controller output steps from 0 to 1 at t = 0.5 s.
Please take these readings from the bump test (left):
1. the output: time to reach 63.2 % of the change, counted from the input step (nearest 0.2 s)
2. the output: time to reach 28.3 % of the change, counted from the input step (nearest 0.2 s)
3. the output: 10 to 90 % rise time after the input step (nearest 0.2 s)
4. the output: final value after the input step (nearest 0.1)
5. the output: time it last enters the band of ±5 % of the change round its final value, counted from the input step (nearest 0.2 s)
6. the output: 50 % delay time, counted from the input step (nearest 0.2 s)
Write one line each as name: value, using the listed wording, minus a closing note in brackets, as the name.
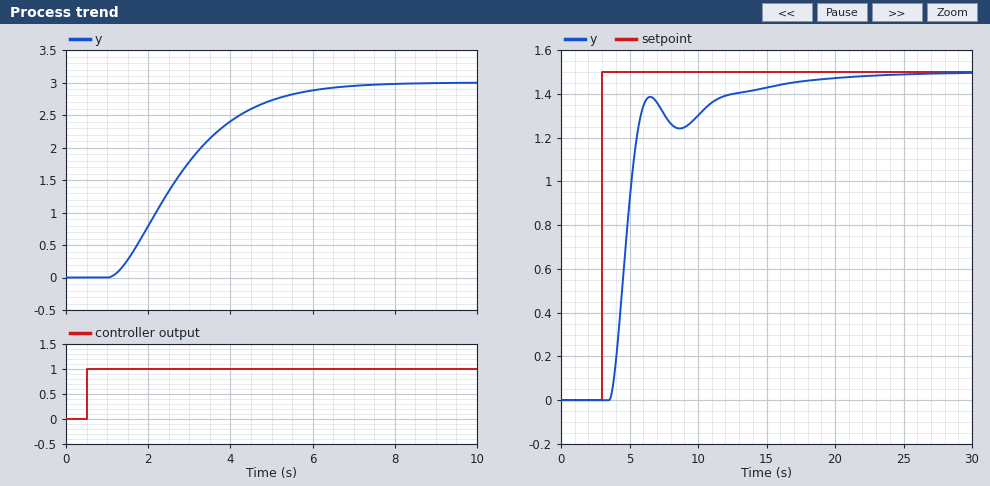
the output: time to reach 63.2 % of the change, counted from the input step: 2.6 s
the output: time to reach 28.3 % of the change, counted from the input step: 1.6 s
the output: 10 to 90 % rise time after the input step: 3.4 s
the output: final value after the input step: 3.0
the output: time it last enters the band of ±5 % of the change round its final value, counted from the input step: 5.2 s
the output: 50 % delay time, counted from the input step: 2.2 s
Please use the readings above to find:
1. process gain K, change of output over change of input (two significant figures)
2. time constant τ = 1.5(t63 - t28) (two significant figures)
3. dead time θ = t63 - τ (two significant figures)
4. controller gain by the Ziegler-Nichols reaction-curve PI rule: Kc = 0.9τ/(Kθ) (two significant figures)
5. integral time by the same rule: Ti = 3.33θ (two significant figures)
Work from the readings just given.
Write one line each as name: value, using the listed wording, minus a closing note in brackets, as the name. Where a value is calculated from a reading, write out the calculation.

process gain K, change of output over change of input: (3 - 0) / 1 = 3.0
time constant τ = 1.5(t63 - t28): 1.5 × (2.6 - 1.6) = 1.5 s
dead time θ = t63 - τ: 2.6 - 1.5 = 1.1 s
controller gain by the Ziegler-Nichols reaction-curve PI rule: Kc = 0.9τ/(Kθ): 0.9 × 1.5 / (3 × 1.1) = 0.41
integral time by the same rule: Ti = 3.33θ: 3.33 × 1.1 = 3.7 s
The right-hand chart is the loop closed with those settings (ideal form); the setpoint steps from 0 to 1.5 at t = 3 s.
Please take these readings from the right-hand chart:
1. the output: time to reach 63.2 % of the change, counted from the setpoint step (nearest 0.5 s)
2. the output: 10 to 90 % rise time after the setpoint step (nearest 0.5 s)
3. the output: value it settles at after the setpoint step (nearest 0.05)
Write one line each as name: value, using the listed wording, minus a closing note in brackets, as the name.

the output: time to reach 63.2 % of the change, counted from the setpoint step: 2.0 s
the output: 10 to 90 % rise time after the setpoint step: 2.0 s
the output: value it settles at after the setpoint step: 1.50
